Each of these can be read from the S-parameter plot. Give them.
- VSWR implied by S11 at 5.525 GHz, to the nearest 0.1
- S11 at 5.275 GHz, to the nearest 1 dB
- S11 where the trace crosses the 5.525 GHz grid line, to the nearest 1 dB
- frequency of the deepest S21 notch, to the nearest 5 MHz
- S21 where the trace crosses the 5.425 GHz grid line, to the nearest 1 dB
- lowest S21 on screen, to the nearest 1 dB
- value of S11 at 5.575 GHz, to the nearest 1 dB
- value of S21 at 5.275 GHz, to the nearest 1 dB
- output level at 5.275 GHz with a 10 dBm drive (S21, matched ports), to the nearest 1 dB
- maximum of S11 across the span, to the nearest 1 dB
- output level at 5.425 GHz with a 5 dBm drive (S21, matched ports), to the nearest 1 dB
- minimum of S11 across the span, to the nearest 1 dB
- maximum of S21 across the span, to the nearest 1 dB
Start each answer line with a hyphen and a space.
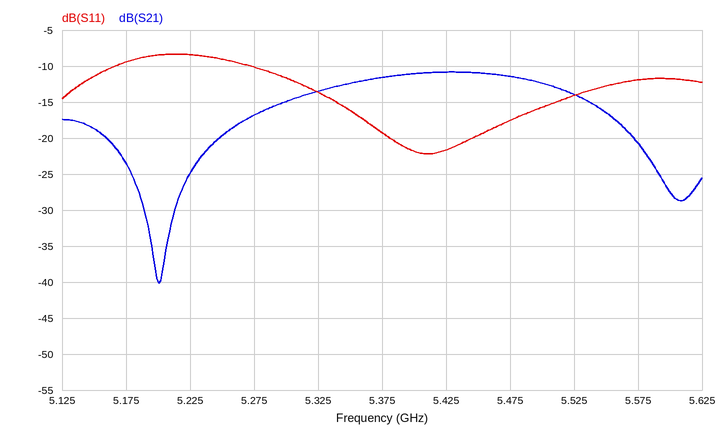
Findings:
- 1.5
- -10 dB
- -14 dB
- 5.200 GHz
- -11 dB
- -40 dB
- -12 dB
- -17 dB
- -7 dBm
- -8 dB
- -6 dBm
- -22 dB
- -11 dB
